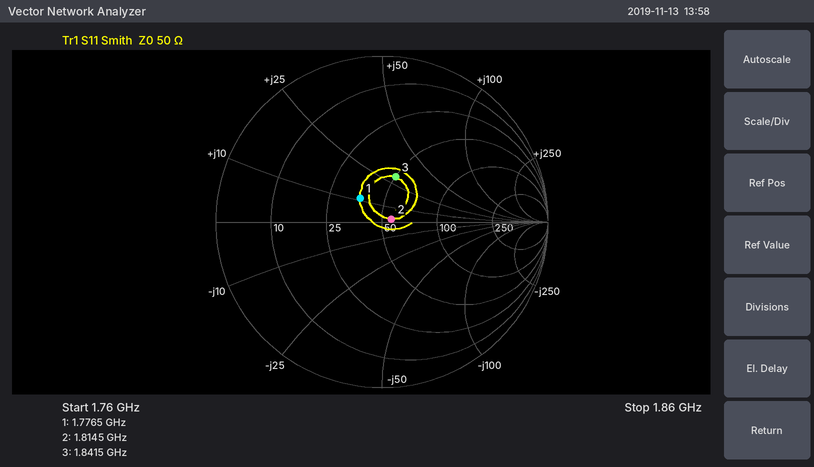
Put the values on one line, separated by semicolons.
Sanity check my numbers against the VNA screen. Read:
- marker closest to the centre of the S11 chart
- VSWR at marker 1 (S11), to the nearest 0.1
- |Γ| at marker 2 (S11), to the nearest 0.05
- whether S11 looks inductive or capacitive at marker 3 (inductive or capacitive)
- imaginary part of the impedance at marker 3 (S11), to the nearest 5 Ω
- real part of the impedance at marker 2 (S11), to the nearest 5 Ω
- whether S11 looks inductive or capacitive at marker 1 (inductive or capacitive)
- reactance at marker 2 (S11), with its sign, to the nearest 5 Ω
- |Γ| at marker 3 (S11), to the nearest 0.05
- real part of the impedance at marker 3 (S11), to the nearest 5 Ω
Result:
marker 2; 1.5; 0.05; inductive; +30 Ω; 55 Ω; inductive; 0 Ω; 0.30; 50 Ω
